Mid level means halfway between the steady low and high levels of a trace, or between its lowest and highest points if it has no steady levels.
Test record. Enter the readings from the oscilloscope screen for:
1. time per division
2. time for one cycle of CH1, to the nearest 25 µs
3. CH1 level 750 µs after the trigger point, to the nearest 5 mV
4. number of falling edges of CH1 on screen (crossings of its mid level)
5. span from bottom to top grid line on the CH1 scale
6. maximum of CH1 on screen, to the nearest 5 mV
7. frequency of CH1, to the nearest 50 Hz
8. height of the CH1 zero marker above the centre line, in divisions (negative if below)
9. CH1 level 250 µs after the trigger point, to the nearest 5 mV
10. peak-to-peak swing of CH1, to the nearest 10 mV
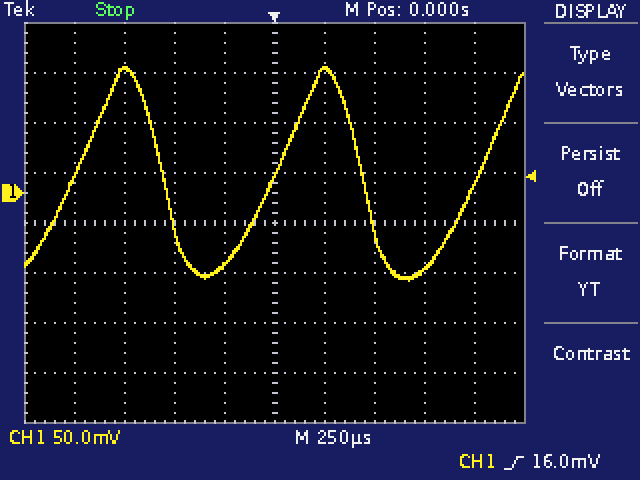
250 µs
1.000 ms
-75 mV
2
400 mV
125 mV
1.00 kHz
+0.6 div
125 mV
210 mV
